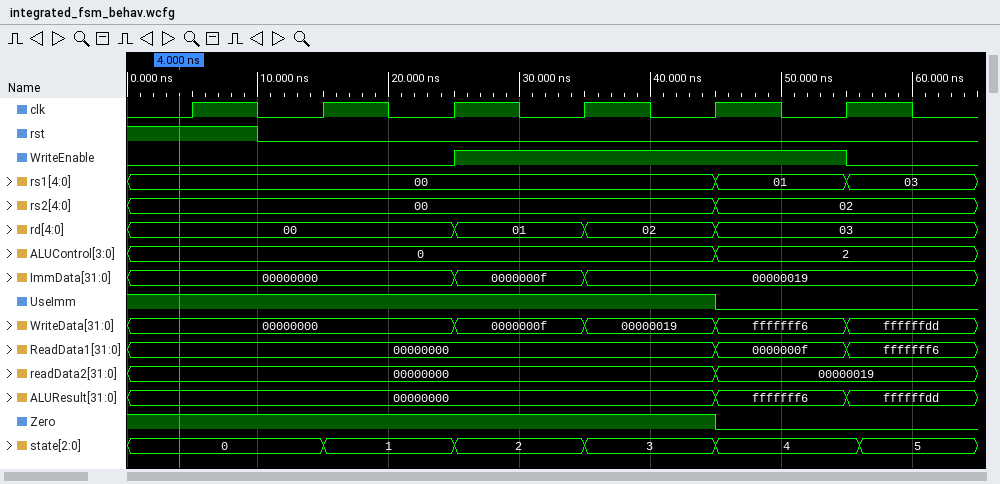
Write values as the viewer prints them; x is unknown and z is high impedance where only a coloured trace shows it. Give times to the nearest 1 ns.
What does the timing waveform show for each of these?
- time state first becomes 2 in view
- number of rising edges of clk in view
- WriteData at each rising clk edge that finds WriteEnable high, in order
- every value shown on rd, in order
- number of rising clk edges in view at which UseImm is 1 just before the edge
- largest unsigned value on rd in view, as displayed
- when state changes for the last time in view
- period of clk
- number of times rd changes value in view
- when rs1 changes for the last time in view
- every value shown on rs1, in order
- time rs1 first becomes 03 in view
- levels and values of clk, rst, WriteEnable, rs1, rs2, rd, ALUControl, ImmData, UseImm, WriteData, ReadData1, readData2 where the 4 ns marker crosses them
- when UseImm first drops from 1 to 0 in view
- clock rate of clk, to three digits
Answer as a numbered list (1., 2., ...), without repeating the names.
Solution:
1. 25 ns
2. 6
3. 0000000f, 00000019, fffffff6
4. 00, 01, 02, 03
5. 5
6. 03
7. 56 ns
8. 10 ns
9. 3
10. 55 ns
11. 00, 01, 03
12. 55 ns
13. clk=0, rst=1, WriteEnable=0, rs1=00, rs2=00, rd=00, ALUControl=0, ImmData=00000000, UseImm=1, WriteData=00000000, ReadData1=00000000, readData2=00000000
14. 45 ns
15. 100 MHz
